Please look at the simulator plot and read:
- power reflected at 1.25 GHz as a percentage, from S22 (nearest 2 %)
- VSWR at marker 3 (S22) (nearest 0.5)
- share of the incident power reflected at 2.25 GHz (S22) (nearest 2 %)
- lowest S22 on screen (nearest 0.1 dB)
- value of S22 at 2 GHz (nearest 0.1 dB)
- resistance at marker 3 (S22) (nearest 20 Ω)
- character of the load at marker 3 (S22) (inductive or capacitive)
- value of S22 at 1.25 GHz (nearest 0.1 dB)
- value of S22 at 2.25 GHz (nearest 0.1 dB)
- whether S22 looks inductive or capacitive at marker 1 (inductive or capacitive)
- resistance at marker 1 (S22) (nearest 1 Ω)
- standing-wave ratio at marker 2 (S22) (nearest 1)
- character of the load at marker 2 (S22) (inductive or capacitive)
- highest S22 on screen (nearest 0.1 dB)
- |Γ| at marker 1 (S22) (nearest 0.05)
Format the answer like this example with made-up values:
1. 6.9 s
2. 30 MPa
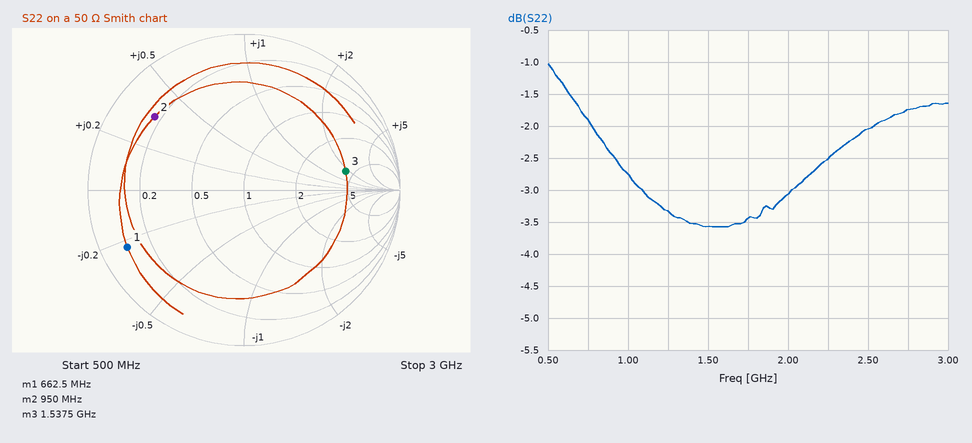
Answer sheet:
1. 46 %
2. 5.0
3. 56 %
4. -3.6 dB
5. -3.1 dB
6. 200 Ω
7. inductive
8. -3.3 dB
9. -2.5 dB
10. capacitive
11. 5 Ω
12. 7
13. inductive
14. -1.0 dB
15. 0.85
